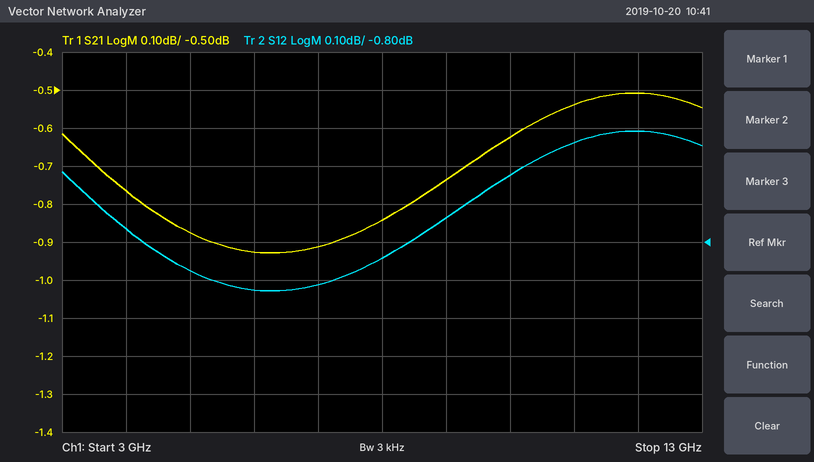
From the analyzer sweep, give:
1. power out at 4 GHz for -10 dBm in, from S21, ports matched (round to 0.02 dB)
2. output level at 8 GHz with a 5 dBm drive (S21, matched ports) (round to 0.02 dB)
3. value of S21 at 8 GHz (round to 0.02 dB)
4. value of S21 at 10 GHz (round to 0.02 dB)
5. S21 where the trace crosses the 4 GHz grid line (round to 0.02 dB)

-10.76 dBm
4.16 dBm
-0.84 dB
-0.62 dB
-0.76 dB
